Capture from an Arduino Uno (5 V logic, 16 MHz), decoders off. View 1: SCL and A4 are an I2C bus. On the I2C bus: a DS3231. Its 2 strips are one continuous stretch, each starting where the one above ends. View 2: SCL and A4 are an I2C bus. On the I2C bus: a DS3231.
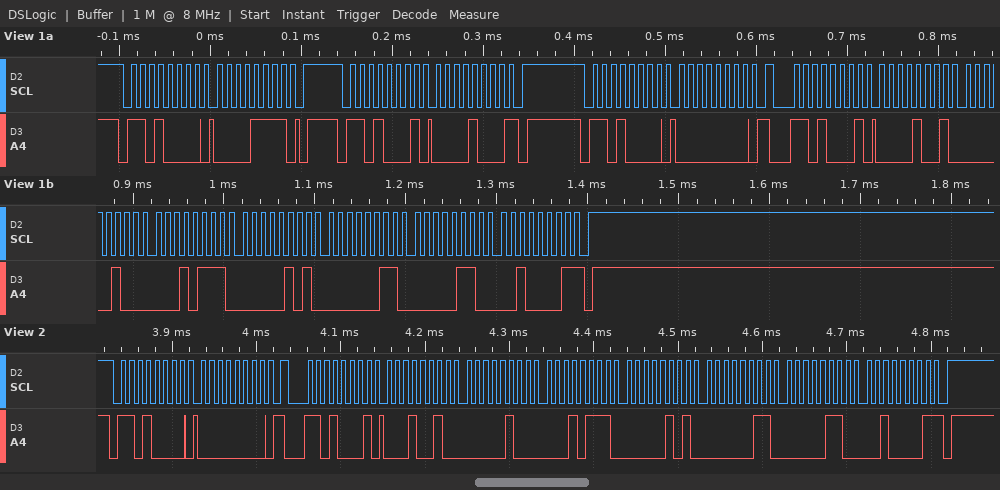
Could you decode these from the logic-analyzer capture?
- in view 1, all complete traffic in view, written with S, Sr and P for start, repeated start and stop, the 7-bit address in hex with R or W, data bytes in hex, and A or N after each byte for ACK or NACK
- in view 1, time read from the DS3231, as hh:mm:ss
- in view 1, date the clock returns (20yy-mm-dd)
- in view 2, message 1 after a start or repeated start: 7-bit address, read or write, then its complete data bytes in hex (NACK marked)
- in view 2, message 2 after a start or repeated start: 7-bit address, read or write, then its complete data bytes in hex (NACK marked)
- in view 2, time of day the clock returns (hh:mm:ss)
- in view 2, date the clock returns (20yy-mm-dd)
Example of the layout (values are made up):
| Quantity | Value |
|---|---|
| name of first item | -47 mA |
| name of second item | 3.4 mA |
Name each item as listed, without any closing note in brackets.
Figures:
| Quantity | Value |
|---|---|
| in view 1, all complete traffic in view, written with S, Sr and P for start, repeated start and stop, the 7-bit address in hex with R or W, data bytes in hex, and A or N after each byte for ACK or NACK | S 68W A 0F A P S 68R A 08 N P S 68W A 00 A Sr 68R A 09 A 04 A 17 A 05 A 03 A 06 A 21 N P |
| in view 1, time read from the DS3231, as hh:mm:ss | 17:04:09 |
| in view 1, date the clock returns | 2021-06-03 |
| in view 2, message 1 after a start or repeated start: 7-bit address, read or write, then its complete data bytes in hex | 0x68 write: 00 |
| in view 2, message 2 after a start or repeated start: 7-bit address, read or write, then its complete data bytes in hex | 0x68 read: 12 04 17 05 03 06 21 NACK |
| in view 2, time of day the clock returns | 17:04:12 |
| in view 2, date the clock returns | 2021-06-03 |
